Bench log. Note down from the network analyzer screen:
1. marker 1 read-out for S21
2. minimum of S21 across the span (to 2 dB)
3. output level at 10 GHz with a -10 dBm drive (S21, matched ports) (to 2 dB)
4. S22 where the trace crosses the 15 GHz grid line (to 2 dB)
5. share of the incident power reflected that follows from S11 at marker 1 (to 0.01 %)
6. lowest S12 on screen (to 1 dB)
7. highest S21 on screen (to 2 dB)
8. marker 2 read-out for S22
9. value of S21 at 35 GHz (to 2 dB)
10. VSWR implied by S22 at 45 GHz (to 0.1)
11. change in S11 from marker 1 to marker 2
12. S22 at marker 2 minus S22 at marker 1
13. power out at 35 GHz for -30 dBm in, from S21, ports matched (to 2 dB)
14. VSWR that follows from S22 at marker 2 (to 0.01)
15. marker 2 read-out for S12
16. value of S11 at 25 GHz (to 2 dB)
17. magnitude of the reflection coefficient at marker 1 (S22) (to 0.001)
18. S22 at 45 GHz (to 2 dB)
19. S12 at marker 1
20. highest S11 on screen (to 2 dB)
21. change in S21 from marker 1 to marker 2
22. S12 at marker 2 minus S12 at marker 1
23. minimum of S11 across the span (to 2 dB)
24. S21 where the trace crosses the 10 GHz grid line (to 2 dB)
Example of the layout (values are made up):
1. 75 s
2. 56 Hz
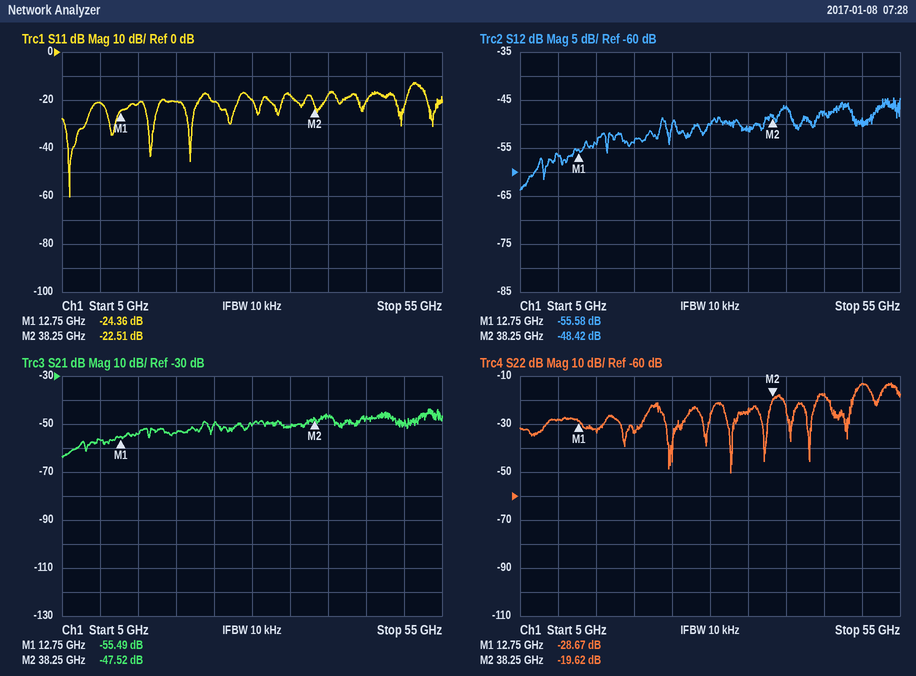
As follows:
1. -55.49 dB
2. -64 dB
3. -66 dBm
4. -32 dB
5. 0.37 %
6. -64 dB
7. -44 dB
8. -19.62 dB
9. -52 dB
10. 1.3
11. 1.85 dB
12. 9.05 dB
13. -82 dBm
14. 1.23
15. -48.42 dB
16. -20 dB
17. 0.037
18. -18 dB
19. -55.58 dB
20. -12 dB
21. 7.97 dB
22. 7.16 dB
23. -60 dB
24. -56 dB
